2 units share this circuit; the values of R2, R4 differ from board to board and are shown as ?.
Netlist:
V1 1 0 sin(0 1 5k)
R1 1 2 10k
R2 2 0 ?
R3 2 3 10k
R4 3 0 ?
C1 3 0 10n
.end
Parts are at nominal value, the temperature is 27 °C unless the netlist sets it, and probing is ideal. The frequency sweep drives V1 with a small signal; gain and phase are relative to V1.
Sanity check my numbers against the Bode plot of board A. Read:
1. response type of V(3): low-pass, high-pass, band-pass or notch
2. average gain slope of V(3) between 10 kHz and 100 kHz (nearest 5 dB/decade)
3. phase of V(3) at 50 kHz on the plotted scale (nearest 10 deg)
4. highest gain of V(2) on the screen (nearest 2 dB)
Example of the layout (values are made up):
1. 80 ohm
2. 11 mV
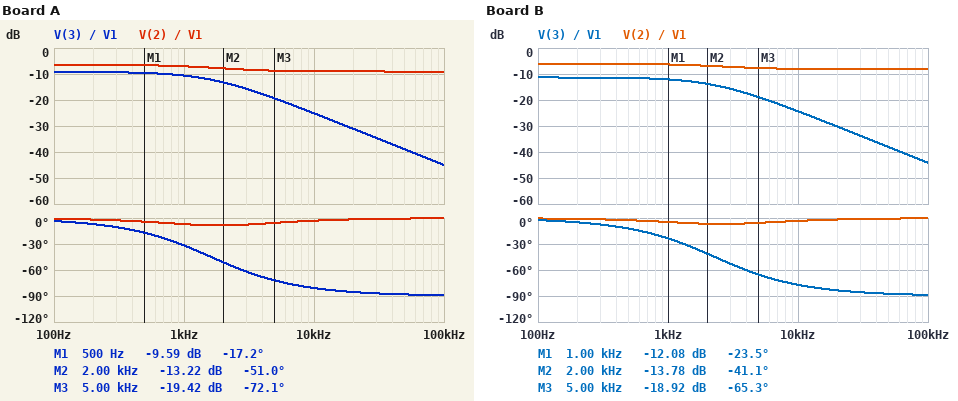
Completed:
1. low-pass
2. -20 dB/decade
3. -90 deg
4. -6 dB
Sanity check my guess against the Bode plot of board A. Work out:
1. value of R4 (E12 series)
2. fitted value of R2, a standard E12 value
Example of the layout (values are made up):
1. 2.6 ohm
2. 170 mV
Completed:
1. 27 kΩ
2. 12 kΩ
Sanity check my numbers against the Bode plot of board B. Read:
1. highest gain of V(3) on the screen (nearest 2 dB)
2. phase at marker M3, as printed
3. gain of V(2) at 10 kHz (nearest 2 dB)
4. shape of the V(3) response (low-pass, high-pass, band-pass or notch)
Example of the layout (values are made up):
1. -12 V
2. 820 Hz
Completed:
1. -12 dB
2. -65.3 deg
3. -8 dB
4. low-pass
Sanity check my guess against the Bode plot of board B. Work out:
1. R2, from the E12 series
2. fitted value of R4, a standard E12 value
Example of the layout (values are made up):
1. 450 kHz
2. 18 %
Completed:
1. 18 kΩ
2. 12 kΩ
